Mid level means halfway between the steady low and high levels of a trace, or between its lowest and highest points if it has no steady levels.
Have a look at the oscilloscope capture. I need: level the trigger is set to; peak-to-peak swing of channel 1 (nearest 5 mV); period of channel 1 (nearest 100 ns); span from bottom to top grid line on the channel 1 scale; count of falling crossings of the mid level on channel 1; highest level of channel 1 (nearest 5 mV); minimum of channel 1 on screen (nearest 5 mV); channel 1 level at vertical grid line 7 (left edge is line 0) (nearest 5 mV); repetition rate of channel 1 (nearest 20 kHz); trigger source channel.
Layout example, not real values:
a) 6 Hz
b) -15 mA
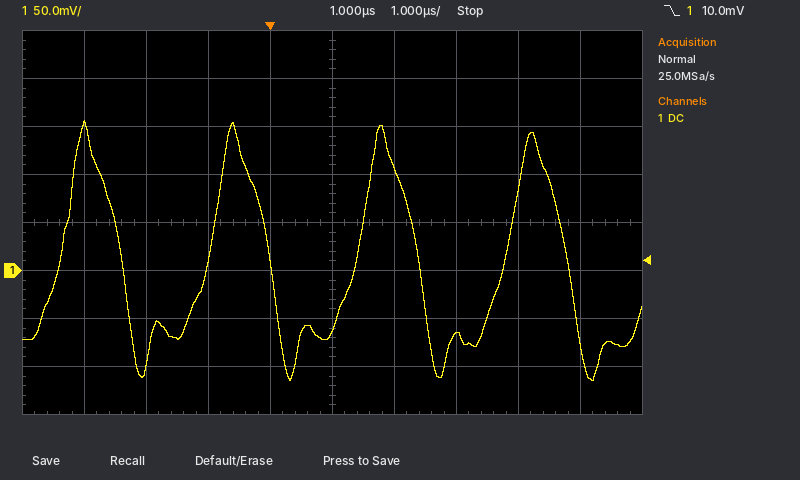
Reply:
a) 10.0 mV
b) 270 mV
c) 2.4 µs
d) 400 mV
e) 4
f) 155 mV
g) -115 mV
h) -65 mV
i) 420 kHz
j) channel 1
